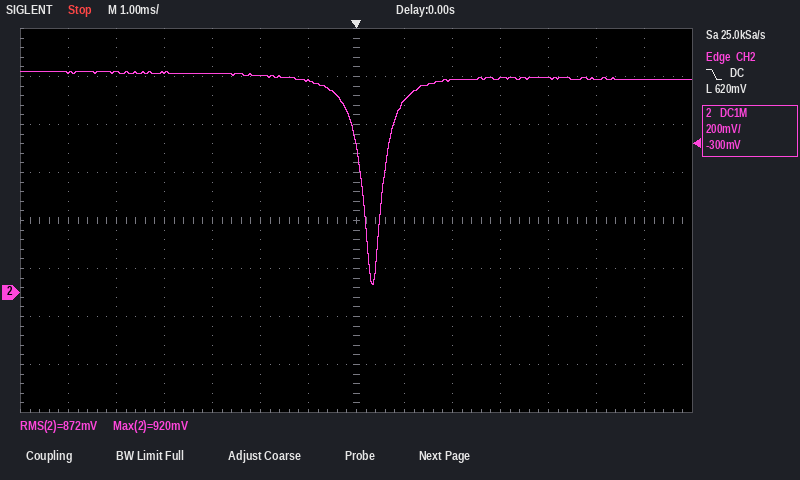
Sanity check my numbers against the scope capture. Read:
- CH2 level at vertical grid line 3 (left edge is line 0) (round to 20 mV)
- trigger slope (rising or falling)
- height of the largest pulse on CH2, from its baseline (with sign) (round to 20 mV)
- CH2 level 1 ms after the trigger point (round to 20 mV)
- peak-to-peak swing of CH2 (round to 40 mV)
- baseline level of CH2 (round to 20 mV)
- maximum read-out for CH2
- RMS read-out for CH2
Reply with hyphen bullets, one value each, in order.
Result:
- 920 mV
- falling
- -860 mV
- 800 mV
- 880 mV
- 900 mV
- 920 mV
- 872 mV
